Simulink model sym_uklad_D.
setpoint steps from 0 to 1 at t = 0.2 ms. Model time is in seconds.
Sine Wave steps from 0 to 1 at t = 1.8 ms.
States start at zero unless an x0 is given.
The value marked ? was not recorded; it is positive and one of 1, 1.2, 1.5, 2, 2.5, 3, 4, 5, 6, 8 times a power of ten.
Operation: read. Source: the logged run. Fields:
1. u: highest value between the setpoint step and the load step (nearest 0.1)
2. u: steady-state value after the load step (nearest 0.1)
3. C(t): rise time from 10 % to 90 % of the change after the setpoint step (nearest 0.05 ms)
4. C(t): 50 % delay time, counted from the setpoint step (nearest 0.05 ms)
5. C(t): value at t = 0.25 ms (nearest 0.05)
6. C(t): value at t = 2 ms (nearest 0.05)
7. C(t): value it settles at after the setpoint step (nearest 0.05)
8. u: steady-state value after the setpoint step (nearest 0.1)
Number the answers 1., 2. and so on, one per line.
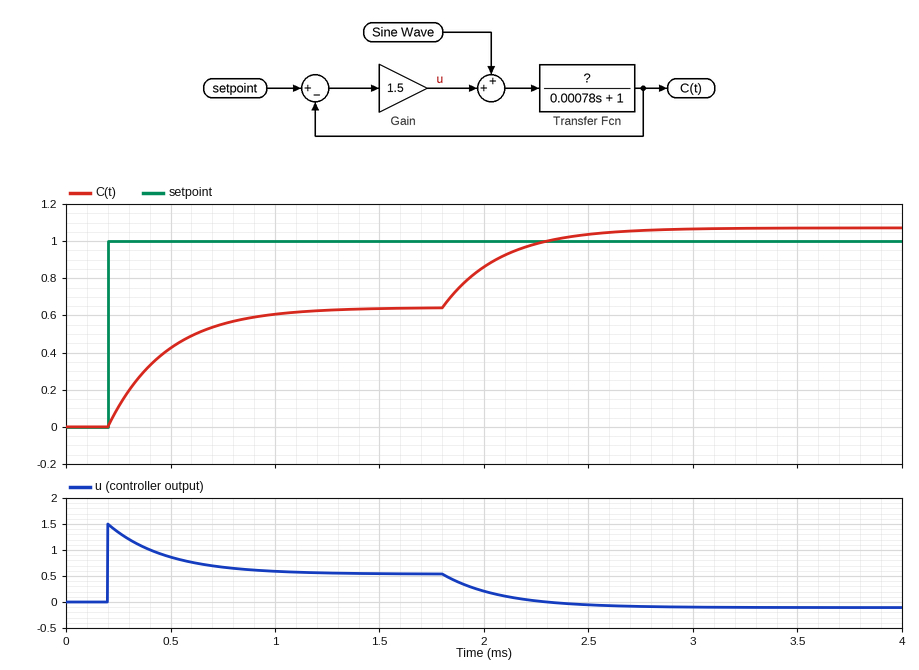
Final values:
1. 1.5
2. -0.1
3. 0.60 ms
4. 0.20 ms
5. 0.10
6. 0.85
7. 0.65
8. 0.5
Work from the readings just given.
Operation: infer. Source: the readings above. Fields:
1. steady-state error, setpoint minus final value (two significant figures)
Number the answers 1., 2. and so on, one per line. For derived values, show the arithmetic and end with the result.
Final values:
1. 1 - 0.65 = 0.35
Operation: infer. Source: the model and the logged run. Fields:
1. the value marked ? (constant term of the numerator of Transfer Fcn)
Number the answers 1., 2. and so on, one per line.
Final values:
1. 1.2
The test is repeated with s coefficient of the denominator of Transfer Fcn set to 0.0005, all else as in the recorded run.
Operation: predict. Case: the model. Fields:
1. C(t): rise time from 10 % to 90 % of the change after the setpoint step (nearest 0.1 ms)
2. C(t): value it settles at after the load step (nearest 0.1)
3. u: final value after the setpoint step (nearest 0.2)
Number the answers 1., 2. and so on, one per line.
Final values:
1. 0.4 ms
2. 1.1
3. 0.6
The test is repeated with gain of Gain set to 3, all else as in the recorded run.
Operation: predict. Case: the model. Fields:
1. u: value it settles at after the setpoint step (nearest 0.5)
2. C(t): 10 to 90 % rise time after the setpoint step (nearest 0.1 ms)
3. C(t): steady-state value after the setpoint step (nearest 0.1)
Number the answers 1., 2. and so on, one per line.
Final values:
1. 0.5
2. 0.4 ms
3. 0.8
